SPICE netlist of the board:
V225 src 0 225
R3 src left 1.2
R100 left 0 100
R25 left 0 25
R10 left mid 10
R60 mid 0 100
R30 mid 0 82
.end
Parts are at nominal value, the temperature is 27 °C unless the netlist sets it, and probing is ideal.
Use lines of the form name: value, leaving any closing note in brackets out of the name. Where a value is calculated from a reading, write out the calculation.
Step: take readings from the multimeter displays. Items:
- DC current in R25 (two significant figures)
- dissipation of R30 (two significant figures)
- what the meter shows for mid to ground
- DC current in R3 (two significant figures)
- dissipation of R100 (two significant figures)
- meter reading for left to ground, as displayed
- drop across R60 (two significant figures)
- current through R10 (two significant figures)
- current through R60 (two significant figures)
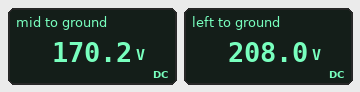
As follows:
DC current in R25: (208 V) / 25 Ω = 8.3 A
dissipation of R30: (170.2 V)^2 / 82 Ω = 350 W
what the meter shows for mid to ground: 170.2 V
DC current in R3: (225 V - 208 V) / 1.2 Ω = 14 A
dissipation of R100: (208 V)^2 / 100 Ω = 430 W
meter reading for left to ground, as displayed: 208.0 V
drop across R60: 170.2 V = 170 V
current through R10: (208 V - 170.2 V) / 10 Ω = 3.8 A
current through R60: (170.2 V) / 100 Ω = 1.7 A
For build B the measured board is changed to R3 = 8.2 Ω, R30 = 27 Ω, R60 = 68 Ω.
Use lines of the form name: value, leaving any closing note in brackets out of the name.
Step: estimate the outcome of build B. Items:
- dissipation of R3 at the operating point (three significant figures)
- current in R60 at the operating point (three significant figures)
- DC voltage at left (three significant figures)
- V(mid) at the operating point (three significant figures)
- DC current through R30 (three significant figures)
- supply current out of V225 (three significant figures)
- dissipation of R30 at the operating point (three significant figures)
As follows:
dissipation of R3 at the operating point: 1.03 kW
current in R60 at the operating point: 1.29 A
DC voltage at left: 133 V
V(mid) at the operating point: 87.8 V
DC current through R30: 3.25 A
supply current out of V225: 11.2 A
dissipation of R30 at the operating point: 285 W
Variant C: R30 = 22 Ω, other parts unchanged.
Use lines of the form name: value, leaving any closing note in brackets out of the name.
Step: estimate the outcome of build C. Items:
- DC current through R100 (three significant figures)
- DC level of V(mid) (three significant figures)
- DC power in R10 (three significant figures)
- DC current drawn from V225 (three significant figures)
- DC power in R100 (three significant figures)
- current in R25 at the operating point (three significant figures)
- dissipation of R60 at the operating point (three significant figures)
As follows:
DC current through R100: 2.04 A
DC level of V(mid): 131 V
DC power in R10: 530 W
DC current drawn from V225: 17.5 A
DC power in R100: 416 W
current in R25 at the operating point: 8.16 A
dissipation of R60 at the operating point: 172 W
